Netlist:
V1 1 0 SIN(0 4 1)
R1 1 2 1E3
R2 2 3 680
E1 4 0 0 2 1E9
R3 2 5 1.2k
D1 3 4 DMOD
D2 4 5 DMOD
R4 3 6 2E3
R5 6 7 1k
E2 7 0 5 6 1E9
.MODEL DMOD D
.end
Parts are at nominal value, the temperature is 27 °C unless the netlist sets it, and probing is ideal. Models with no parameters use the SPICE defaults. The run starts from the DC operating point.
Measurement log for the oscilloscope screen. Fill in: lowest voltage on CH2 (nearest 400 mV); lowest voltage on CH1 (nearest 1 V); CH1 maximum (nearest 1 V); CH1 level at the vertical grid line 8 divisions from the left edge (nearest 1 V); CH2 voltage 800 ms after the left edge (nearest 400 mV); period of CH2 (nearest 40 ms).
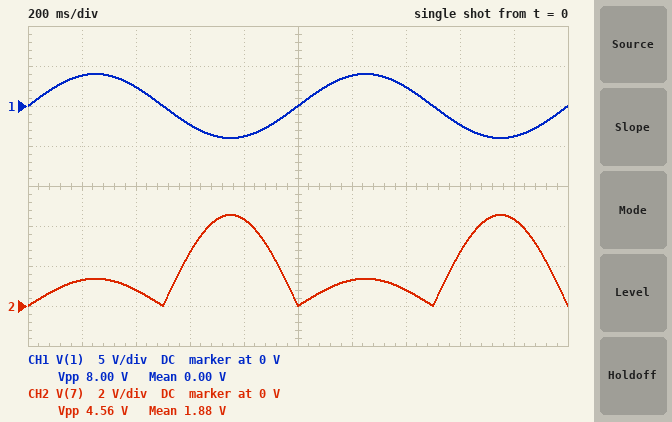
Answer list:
0 V
-4 V
4 V
-2 V
4.4 V
1.00 s
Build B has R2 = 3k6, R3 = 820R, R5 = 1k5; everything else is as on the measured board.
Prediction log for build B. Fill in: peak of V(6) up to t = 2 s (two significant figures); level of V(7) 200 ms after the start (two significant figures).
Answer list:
2.9 V
10 V
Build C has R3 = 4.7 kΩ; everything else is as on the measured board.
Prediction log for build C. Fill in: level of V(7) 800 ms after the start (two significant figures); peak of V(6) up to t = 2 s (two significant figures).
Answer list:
8.9 V
6.8 V
